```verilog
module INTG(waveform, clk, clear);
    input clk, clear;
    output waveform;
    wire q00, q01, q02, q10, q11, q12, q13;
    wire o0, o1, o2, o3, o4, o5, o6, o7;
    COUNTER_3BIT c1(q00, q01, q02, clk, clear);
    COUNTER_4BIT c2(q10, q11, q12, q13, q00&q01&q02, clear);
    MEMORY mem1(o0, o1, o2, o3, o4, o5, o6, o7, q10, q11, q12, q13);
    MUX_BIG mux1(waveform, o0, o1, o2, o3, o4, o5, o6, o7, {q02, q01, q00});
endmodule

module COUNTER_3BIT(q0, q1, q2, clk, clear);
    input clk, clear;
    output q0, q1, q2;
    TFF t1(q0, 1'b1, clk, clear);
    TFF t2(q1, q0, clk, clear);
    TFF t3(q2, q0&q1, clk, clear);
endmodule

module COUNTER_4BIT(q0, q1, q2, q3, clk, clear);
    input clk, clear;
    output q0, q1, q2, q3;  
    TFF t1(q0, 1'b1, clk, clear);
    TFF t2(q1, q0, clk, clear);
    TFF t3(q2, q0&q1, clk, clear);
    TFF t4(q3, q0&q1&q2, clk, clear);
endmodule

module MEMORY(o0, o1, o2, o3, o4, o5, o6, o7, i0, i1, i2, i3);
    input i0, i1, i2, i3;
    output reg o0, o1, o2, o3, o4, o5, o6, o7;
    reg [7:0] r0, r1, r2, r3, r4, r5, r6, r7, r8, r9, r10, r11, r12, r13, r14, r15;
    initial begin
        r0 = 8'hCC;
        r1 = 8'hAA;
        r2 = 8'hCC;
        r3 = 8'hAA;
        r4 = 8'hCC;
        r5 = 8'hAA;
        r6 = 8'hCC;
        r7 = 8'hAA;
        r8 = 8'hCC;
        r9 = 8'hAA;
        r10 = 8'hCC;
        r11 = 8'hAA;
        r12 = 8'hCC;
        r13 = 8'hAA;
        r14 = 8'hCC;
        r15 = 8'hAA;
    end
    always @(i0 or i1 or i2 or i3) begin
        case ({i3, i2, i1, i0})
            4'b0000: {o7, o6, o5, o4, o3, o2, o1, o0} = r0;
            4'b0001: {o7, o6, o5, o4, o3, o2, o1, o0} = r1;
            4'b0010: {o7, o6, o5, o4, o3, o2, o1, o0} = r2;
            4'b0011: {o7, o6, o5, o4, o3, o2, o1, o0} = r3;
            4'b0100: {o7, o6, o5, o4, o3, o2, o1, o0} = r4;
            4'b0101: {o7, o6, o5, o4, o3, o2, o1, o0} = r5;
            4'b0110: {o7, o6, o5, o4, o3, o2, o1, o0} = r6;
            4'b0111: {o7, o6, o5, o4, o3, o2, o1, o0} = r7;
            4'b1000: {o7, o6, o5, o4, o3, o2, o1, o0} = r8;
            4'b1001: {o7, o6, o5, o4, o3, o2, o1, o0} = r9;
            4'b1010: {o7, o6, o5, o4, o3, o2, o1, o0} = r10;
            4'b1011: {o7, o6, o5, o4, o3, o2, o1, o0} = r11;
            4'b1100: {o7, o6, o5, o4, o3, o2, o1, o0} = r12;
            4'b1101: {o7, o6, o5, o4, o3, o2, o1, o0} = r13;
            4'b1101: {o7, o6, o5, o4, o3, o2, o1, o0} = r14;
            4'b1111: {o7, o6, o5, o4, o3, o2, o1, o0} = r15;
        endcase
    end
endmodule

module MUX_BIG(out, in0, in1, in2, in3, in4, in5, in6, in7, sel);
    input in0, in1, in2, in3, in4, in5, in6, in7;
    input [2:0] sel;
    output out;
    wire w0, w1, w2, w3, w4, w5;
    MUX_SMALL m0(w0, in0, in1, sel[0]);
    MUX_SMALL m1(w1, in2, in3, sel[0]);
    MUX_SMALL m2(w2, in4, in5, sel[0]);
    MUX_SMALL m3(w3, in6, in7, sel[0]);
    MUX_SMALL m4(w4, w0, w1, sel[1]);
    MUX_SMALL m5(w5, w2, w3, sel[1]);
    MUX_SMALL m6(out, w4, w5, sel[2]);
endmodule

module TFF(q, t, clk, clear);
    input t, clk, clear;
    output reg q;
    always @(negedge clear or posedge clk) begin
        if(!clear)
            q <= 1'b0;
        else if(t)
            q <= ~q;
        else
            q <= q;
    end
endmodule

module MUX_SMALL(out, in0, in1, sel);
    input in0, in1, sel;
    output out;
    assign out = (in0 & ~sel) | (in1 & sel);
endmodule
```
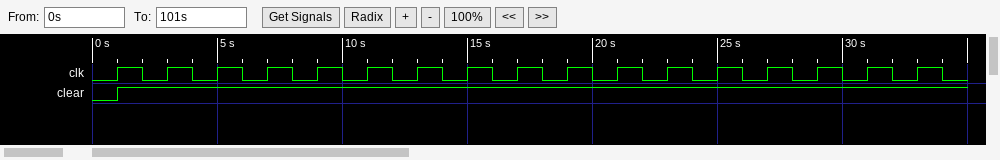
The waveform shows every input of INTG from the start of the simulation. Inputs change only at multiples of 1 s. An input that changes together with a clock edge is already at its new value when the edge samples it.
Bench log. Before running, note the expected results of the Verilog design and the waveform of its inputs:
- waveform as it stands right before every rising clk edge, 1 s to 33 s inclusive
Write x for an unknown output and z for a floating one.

0 0 1 1 0 1 0 1 0 0 1 1 0 1 0 1 0
